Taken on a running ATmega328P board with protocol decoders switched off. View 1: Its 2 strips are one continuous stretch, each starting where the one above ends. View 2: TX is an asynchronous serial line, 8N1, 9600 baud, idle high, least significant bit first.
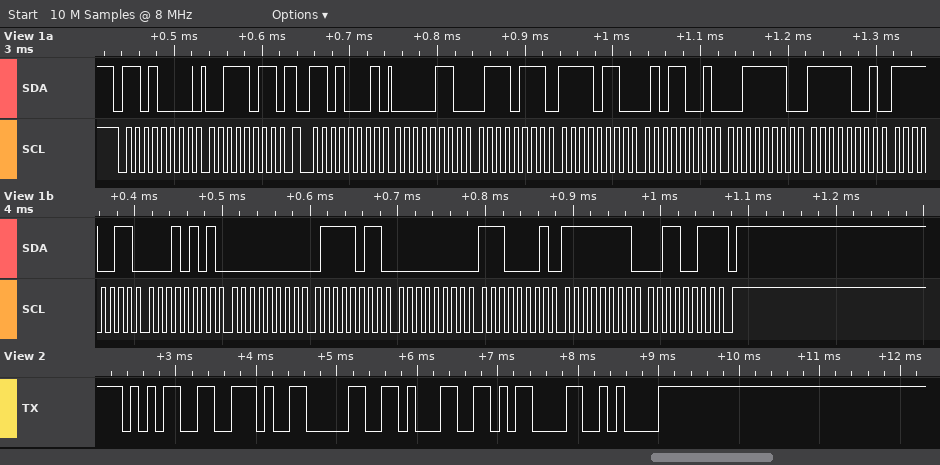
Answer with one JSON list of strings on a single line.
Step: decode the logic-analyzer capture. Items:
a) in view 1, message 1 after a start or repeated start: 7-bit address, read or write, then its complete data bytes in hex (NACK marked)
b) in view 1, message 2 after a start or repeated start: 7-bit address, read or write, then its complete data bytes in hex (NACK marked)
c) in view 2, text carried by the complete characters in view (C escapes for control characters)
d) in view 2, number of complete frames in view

["0x68 write: 3B", "0x68 read: 06 77 F6 59 3E F9 F3 15 00 7B 00 E1 FF 33 NACK", "\"5.01\\r\\n\"", "6"]
